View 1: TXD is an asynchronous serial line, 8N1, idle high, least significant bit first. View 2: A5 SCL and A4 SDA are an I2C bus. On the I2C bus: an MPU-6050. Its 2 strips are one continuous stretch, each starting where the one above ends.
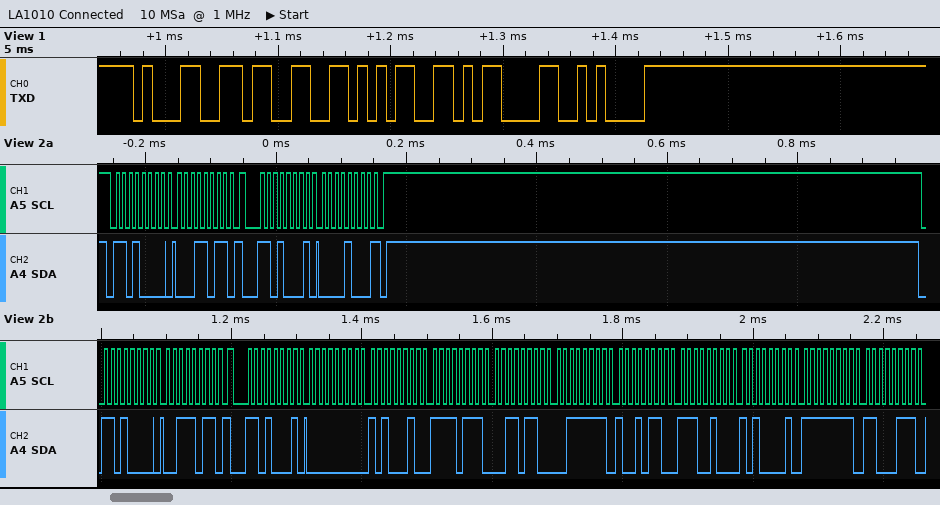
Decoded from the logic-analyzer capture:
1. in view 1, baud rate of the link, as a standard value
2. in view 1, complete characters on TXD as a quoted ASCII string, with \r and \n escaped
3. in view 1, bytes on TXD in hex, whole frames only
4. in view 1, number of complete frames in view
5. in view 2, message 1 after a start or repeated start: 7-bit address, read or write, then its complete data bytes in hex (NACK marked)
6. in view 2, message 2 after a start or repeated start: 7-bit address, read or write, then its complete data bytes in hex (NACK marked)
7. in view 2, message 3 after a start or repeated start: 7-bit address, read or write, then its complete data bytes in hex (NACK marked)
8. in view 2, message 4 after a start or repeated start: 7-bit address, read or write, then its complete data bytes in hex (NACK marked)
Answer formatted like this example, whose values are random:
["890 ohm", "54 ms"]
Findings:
["115200 baud", "\"135\\r\\n\"", "31 33 35 0D 0A", "5", "0x68 write: 1B", "0x68 read: 08 NACK", "0x68 write: 3B", "0x68 read: 00 A2 F7 36 3F 96 E4 A1 FF C7"]
